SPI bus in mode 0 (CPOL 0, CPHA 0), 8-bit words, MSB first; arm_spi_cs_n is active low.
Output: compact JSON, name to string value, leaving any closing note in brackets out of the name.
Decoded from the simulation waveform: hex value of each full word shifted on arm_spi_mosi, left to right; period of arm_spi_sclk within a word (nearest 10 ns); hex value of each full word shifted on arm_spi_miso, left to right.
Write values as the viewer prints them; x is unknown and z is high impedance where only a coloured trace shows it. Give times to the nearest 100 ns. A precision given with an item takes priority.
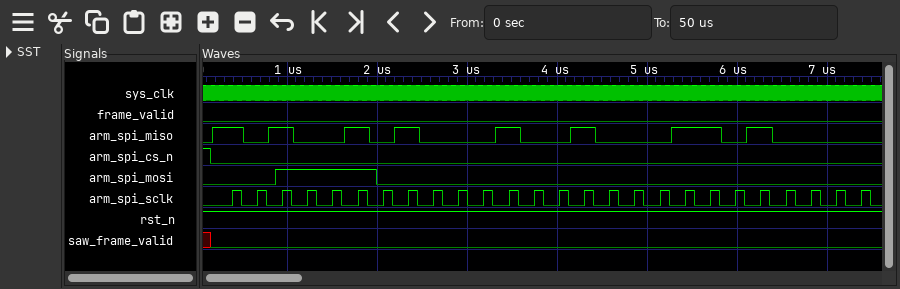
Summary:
{"hex value of each full word shifted on arm_spi_mosi, left to right": "3C, 00, 00", "period of arm_spi_sclk within a word": "280 ns", "hex value of each full word shifted on arm_spi_miso, left to right": "A5, 12, 34"}
